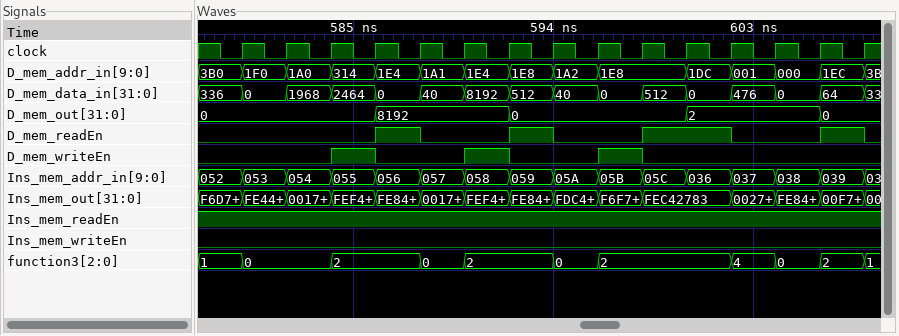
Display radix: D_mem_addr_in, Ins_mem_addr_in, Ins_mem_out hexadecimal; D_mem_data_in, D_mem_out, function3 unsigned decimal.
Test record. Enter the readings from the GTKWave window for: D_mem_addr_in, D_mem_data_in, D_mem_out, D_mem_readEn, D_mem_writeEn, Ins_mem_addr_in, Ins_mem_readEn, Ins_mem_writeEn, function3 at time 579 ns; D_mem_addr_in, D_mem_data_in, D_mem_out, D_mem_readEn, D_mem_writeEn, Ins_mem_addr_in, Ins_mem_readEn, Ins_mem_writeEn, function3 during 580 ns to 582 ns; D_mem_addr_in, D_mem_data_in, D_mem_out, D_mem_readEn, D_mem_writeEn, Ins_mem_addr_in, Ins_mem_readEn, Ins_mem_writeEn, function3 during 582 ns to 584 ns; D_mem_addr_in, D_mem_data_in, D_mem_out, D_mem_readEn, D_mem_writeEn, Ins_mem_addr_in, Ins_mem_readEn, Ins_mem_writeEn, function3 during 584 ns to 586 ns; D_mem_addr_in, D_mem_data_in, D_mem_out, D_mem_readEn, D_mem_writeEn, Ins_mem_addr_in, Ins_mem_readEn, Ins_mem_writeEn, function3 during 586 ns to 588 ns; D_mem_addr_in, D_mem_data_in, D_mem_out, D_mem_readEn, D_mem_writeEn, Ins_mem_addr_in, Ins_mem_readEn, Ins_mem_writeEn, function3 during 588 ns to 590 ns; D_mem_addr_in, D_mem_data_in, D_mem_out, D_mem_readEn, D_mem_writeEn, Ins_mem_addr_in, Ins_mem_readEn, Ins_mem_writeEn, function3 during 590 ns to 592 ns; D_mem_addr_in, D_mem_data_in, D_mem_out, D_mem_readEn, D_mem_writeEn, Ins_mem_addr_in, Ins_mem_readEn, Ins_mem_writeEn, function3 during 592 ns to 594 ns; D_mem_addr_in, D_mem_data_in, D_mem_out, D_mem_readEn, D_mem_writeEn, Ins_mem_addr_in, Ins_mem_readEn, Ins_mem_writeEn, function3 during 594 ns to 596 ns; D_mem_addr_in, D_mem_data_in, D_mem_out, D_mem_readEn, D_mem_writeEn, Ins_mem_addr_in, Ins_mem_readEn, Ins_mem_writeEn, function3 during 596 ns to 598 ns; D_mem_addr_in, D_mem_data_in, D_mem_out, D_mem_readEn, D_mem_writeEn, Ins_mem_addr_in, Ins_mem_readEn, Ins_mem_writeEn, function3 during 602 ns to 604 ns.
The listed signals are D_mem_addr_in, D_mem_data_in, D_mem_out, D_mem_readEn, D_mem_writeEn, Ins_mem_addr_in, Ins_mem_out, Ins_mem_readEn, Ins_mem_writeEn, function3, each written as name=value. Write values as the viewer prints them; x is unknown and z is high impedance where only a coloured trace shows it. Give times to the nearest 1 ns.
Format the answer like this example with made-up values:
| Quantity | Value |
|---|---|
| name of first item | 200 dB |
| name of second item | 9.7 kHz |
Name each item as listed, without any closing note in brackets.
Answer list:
| Quantity | Value |
|---|---|
| D_mem_addr_in, D_mem_data_in, D_mem_out, D_mem_readEn, D_mem_writeEn, Ins_mem_addr_in, Ins_mem_readEn, Ins_mem_writeEn, function3 at time 579 ns | D_mem_addr_in=3B0, D_mem_data_in=336, D_mem_out=0, D_mem_readEn=0, D_mem_writeEn=0, Ins_mem_addr_in=052, Ins_mem_readEn=1, Ins_mem_writeEn=0, function3=1 |
| D_mem_addr_in, D_mem_data_in, D_mem_out, D_mem_readEn, D_mem_writeEn, Ins_mem_addr_in, Ins_mem_readEn, Ins_mem_writeEn, function3 during 580 ns to 582 ns | D_mem_addr_in=1F0, D_mem_data_in=0, D_mem_out=0, D_mem_readEn=0, D_mem_writeEn=0, Ins_mem_addr_in=053, Ins_mem_readEn=1, Ins_mem_writeEn=0, function3=0 |
| D_mem_addr_in, D_mem_data_in, D_mem_out, D_mem_readEn, D_mem_writeEn, Ins_mem_addr_in, Ins_mem_readEn, Ins_mem_writeEn, function3 during 582 ns to 584 ns | D_mem_addr_in=1A0, D_mem_data_in=1968, D_mem_out=0, D_mem_readEn=0, D_mem_writeEn=0, Ins_mem_addr_in=054, Ins_mem_readEn=1, Ins_mem_writeEn=0, function3=0 |
| D_mem_addr_in, D_mem_data_in, D_mem_out, D_mem_readEn, D_mem_writeEn, Ins_mem_addr_in, Ins_mem_readEn, Ins_mem_writeEn, function3 during 584 ns to 586 ns | D_mem_addr_in=314, D_mem_data_in=2464, D_mem_out=0, D_mem_readEn=0, D_mem_writeEn=1, Ins_mem_addr_in=055, Ins_mem_readEn=1, Ins_mem_writeEn=0, function3=2 |
| D_mem_addr_in, D_mem_data_in, D_mem_out, D_mem_readEn, D_mem_writeEn, Ins_mem_addr_in, Ins_mem_readEn, Ins_mem_writeEn, function3 during 586 ns to 588 ns | D_mem_addr_in=1E4, D_mem_data_in=0, D_mem_out=8192, D_mem_readEn=1, D_mem_writeEn=0, Ins_mem_addr_in=056, Ins_mem_readEn=1, Ins_mem_writeEn=0, function3=2 |
| D_mem_addr_in, D_mem_data_in, D_mem_out, D_mem_readEn, D_mem_writeEn, Ins_mem_addr_in, Ins_mem_readEn, Ins_mem_writeEn, function3 during 588 ns to 590 ns | D_mem_addr_in=1A1, D_mem_data_in=40, D_mem_out=8192, D_mem_readEn=0, D_mem_writeEn=0, Ins_mem_addr_in=057, Ins_mem_readEn=1, Ins_mem_writeEn=0, function3=0 |
| D_mem_addr_in, D_mem_data_in, D_mem_out, D_mem_readEn, D_mem_writeEn, Ins_mem_addr_in, Ins_mem_readEn, Ins_mem_writeEn, function3 during 590 ns to 592 ns | D_mem_addr_in=1E4, D_mem_data_in=8192, D_mem_out=8192, D_mem_readEn=0, D_mem_writeEn=1, Ins_mem_addr_in=058, Ins_mem_readEn=1, Ins_mem_writeEn=0, function3=2 |
| D_mem_addr_in, D_mem_data_in, D_mem_out, D_mem_readEn, D_mem_writeEn, Ins_mem_addr_in, Ins_mem_readEn, Ins_mem_writeEn, function3 during 592 ns to 594 ns | D_mem_addr_in=1E8, D_mem_data_in=512, D_mem_out=0, D_mem_readEn=1, D_mem_writeEn=0, Ins_mem_addr_in=059, Ins_mem_readEn=1, Ins_mem_writeEn=0, function3=2 |
| D_mem_addr_in, D_mem_data_in, D_mem_out, D_mem_readEn, D_mem_writeEn, Ins_mem_addr_in, Ins_mem_readEn, Ins_mem_writeEn, function3 during 594 ns to 596 ns | D_mem_addr_in=1A2, D_mem_data_in=40, D_mem_out=0, D_mem_readEn=0, D_mem_writeEn=0, Ins_mem_addr_in=05A, Ins_mem_readEn=1, Ins_mem_writeEn=0, function3=0 |
| D_mem_addr_in, D_mem_data_in, D_mem_out, D_mem_readEn, D_mem_writeEn, Ins_mem_addr_in, Ins_mem_readEn, Ins_mem_writeEn, function3 during 596 ns to 598 ns | D_mem_addr_in=1E8, D_mem_data_in=0, D_mem_out=0, D_mem_readEn=0, D_mem_writeEn=1, Ins_mem_addr_in=05B, Ins_mem_readEn=1, Ins_mem_writeEn=0, function3=2 |
| D_mem_addr_in, D_mem_data_in, D_mem_out, D_mem_readEn, D_mem_writeEn, Ins_mem_addr_in, Ins_mem_readEn, Ins_mem_writeEn, function3 during 602 ns to 604 ns | D_mem_addr_in=001, D_mem_data_in=476, D_mem_out=2, D_mem_readEn=0, D_mem_writeEn=0, Ins_mem_addr_in=037, Ins_mem_readEn=1, Ins_mem_writeEn=0, function3=4 |
